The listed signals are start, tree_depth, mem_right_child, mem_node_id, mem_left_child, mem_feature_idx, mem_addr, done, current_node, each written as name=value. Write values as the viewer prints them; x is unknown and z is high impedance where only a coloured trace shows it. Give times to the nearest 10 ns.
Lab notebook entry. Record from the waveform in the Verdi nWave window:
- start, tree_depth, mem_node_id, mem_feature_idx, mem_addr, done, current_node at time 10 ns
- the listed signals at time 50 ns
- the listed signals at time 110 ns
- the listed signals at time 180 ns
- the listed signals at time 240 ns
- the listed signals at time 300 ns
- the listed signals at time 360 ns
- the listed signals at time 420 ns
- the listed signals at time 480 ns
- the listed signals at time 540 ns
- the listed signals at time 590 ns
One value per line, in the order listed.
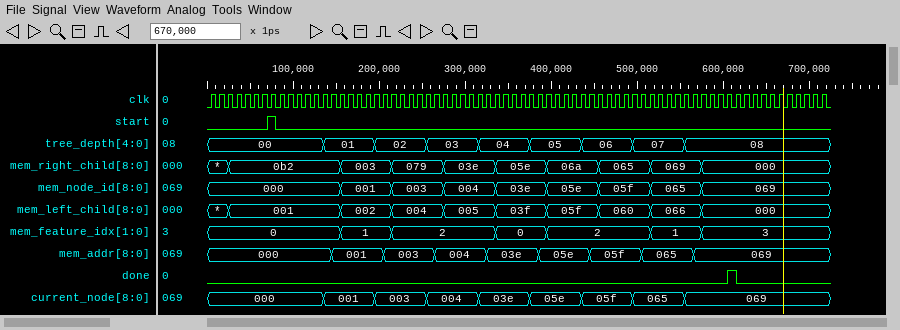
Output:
start=0, tree_depth=00, mem_node_id=000, mem_feature_idx=0, mem_addr=000, done=0, current_node=000
start=0, tree_depth=00, mem_right_child=0b2, mem_node_id=000, mem_left_child=001, mem_feature_idx=0, mem_addr=000, done=0, current_node=000
start=0, tree_depth=00, mem_right_child=0b2, mem_node_id=000, mem_left_child=001, mem_feature_idx=0, mem_addr=000, done=0, current_node=000
start=0, tree_depth=01, mem_right_child=003, mem_node_id=001, mem_left_child=002, mem_feature_idx=1, mem_addr=001, done=0, current_node=001
start=0, tree_depth=02, mem_right_child=079, mem_node_id=003, mem_left_child=004, mem_feature_idx=2, mem_addr=003, done=0, current_node=003
start=0, tree_depth=03, mem_right_child=03e, mem_node_id=004, mem_left_child=005, mem_feature_idx=2, mem_addr=004, done=0, current_node=004
start=0, tree_depth=04, mem_right_child=05e, mem_node_id=03e, mem_left_child=03f, mem_feature_idx=0, mem_addr=03e, done=0, current_node=03e
start=0, tree_depth=05, mem_right_child=06a, mem_node_id=05e, mem_left_child=05f, mem_feature_idx=2, mem_addr=05e, done=0, current_node=05e
start=0, tree_depth=06, mem_right_child=065, mem_node_id=05f, mem_left_child=060, mem_feature_idx=2, mem_addr=05f, done=0, current_node=05f
start=0, tree_depth=07, mem_right_child=069, mem_node_id=065, mem_left_child=066, mem_feature_idx=1, mem_addr=065, done=0, current_node=065
start=0, tree_depth=08, mem_right_child=000, mem_node_id=069, mem_left_child=000, mem_feature_idx=3, mem_addr=069, done=0, current_node=069
